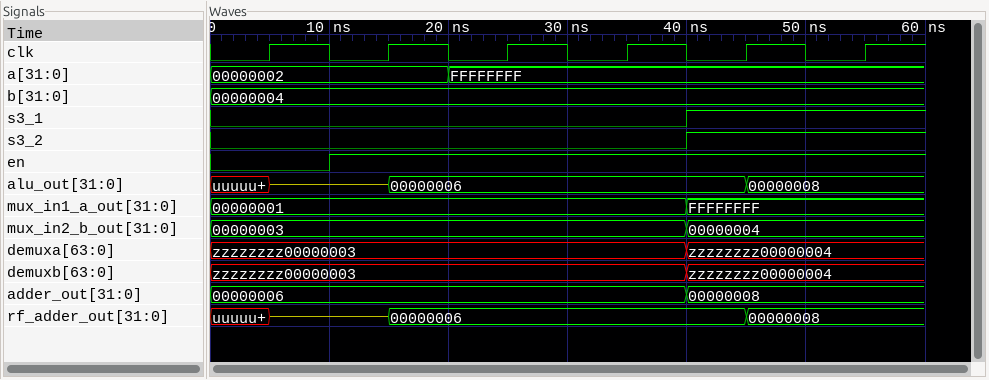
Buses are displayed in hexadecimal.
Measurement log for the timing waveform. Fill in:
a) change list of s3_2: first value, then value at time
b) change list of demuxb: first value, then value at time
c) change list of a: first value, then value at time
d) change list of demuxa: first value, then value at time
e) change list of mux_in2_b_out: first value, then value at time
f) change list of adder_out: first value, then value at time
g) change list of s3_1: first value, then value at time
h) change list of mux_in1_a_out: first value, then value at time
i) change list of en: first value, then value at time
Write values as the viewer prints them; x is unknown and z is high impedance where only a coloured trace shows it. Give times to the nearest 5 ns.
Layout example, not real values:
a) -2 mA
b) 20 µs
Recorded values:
a) 0, 1 at 40 ns
b) zzzzzzzz00000003, zzzzzzzz00000004 at 40 ns
c) 00000002, FFFFFFFF at 20 ns
d) zzzzzzzz00000003, zzzzzzzz00000004 at 40 ns
e) 00000003, 00000004 at 40 ns
f) 00000006, 00000008 at 40 ns
g) 0, 1 at 40 ns
h) 00000001, FFFFFFFF at 40 ns
i) 0, 1 at 10 ns
